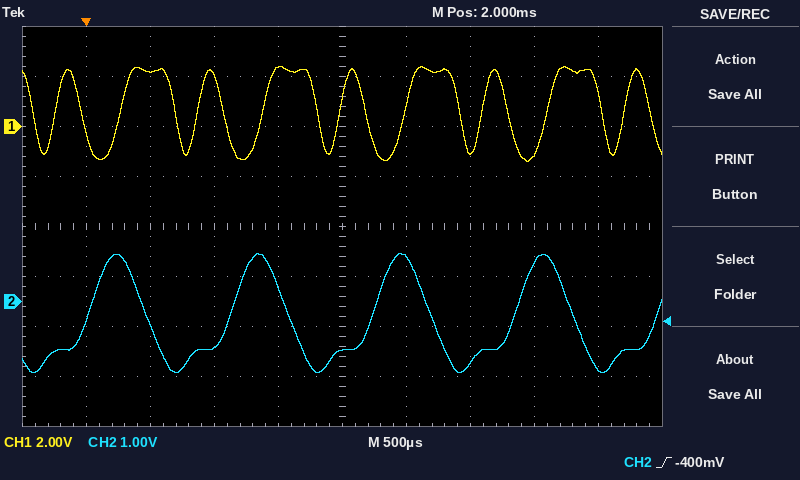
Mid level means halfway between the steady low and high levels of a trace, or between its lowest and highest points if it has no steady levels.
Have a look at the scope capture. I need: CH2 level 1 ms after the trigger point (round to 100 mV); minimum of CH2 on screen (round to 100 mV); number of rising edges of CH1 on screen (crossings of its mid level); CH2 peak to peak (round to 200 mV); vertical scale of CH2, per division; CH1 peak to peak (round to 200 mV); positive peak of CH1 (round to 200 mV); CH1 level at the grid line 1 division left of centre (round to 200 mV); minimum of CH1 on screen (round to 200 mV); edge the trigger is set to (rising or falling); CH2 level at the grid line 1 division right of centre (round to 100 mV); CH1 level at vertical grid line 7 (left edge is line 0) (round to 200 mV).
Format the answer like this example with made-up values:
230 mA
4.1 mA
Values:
-900 mV
-1.4 V
9
2.4 V
1 V
3.8 V
2.4 V
2.4 V
-1.4 V
rising
900 mV
-1.0 V
